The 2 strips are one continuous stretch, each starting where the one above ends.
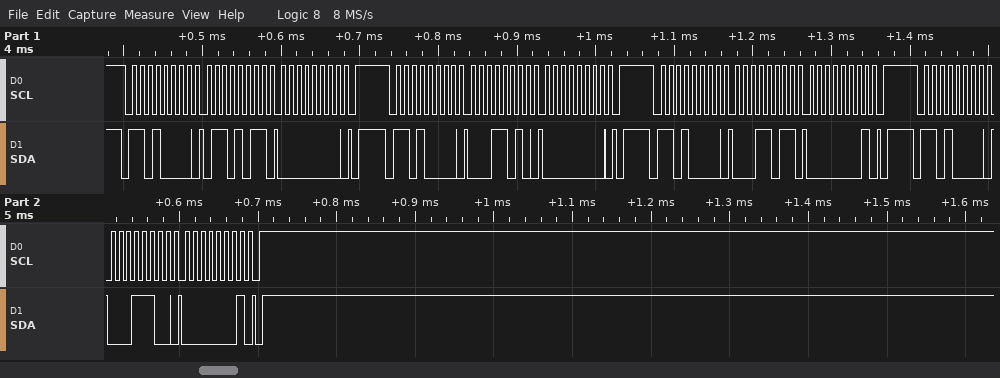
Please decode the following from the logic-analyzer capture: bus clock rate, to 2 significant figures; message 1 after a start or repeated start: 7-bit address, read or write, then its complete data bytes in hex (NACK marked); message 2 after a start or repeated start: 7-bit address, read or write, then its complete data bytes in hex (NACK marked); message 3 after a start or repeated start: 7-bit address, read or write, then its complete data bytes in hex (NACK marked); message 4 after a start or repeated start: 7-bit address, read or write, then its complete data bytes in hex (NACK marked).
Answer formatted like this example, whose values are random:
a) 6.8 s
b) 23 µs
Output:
a) 100 kHz
b) 0x68 write: 6B 00
c) 0x68 write: 1A 00
d) 0x68 write: 1B 01
e) 0x68 write: 1C 01
